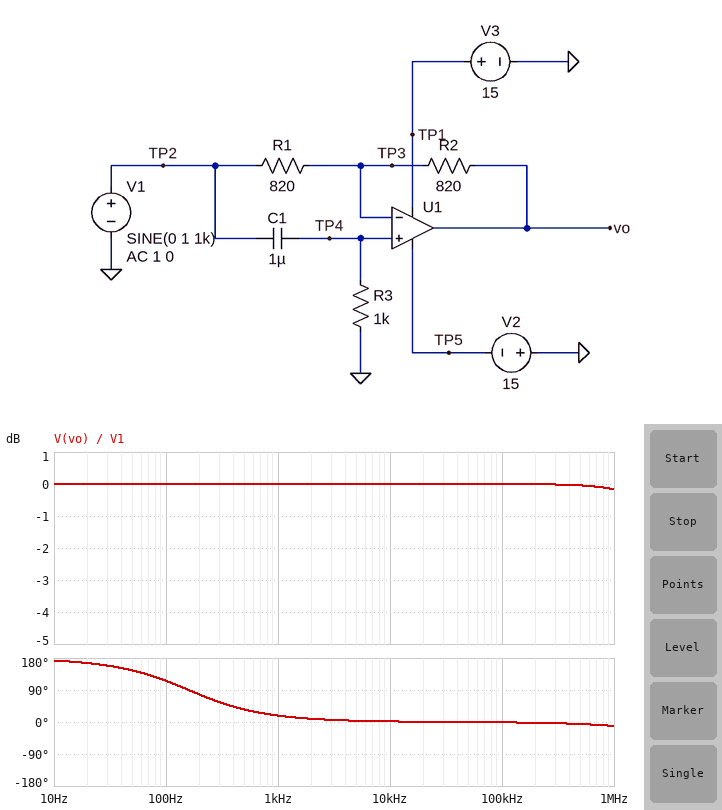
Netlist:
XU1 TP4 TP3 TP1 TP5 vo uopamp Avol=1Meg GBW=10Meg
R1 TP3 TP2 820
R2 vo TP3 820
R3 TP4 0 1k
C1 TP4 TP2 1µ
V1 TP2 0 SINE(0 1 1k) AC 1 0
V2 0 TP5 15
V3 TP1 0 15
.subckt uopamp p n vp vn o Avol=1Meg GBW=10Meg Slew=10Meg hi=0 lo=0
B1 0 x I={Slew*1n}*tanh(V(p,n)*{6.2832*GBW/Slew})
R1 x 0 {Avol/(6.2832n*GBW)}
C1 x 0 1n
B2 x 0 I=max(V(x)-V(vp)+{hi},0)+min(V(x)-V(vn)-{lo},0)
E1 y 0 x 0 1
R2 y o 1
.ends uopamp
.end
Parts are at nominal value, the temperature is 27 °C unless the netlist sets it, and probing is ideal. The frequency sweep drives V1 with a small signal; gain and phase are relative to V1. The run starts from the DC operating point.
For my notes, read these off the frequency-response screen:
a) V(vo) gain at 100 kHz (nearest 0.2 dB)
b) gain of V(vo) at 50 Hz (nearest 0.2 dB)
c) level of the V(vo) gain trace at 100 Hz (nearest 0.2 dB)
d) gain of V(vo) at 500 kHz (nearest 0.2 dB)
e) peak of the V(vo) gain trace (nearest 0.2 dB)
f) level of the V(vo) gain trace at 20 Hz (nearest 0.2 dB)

0 dB
0 dB
0 dB
0 dB
0 dB
0 dB
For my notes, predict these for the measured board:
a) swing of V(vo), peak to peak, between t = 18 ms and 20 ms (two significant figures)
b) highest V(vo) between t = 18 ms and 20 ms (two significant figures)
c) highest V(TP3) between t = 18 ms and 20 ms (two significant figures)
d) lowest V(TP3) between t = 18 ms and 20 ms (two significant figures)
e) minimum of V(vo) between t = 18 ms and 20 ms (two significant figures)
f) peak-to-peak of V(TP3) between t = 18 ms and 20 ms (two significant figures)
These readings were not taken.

2.0 V
1.0 V
990 mV
-990 mV
-1.0 V
2.0 V
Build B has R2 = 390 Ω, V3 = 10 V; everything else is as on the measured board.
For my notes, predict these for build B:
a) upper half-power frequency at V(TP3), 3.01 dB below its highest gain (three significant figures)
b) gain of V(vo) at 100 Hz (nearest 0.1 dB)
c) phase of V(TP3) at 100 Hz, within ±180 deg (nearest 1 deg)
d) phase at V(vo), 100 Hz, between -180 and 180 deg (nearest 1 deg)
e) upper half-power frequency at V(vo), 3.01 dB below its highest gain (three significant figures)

7.61 MHz
-3.5 dB
58 deg
95 deg
6.77 MHz
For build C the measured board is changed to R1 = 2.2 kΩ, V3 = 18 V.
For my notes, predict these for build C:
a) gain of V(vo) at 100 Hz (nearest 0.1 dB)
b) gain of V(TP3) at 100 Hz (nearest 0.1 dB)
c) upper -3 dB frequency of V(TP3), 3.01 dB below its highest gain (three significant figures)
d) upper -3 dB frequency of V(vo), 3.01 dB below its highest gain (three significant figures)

-4.2 dB
-5.5 dB
7.89 MHz
7.28 MHz
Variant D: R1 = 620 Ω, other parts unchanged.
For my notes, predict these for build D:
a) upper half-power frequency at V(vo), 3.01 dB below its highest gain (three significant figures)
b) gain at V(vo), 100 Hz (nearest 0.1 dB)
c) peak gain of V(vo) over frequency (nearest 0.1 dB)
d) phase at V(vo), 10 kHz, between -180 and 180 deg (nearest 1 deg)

1.63 MHz
1.9 dB
2.4 dB
2 deg
